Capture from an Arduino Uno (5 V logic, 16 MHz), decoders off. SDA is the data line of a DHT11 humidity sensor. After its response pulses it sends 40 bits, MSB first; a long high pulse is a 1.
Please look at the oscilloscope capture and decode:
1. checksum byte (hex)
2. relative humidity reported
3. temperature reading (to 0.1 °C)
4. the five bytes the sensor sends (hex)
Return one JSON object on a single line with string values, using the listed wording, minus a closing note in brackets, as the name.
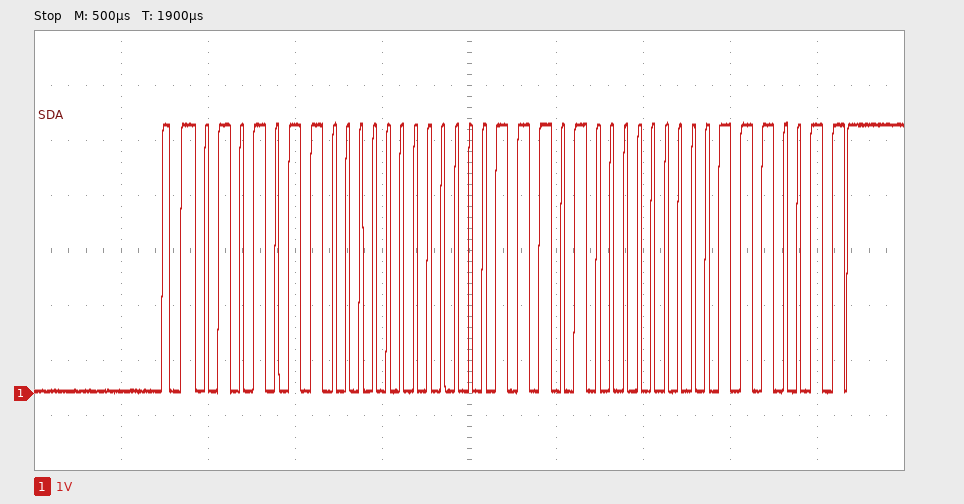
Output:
{"checksum byte": "0x73", "relative humidity reported": "86 %", "temperature reading": "29.0 °C", "the five bytes the sensor sends": "56 00 1D 00 73"}
